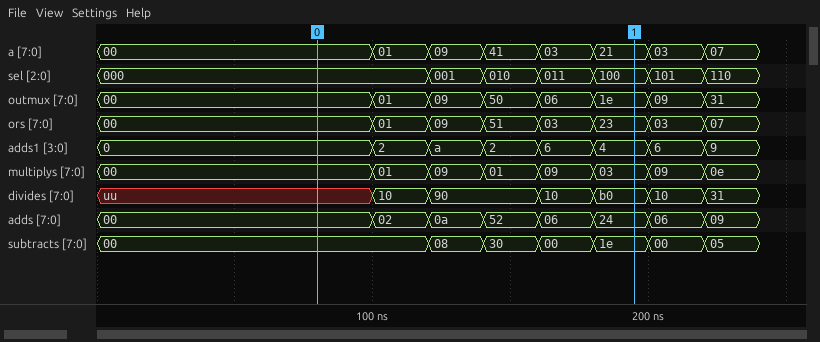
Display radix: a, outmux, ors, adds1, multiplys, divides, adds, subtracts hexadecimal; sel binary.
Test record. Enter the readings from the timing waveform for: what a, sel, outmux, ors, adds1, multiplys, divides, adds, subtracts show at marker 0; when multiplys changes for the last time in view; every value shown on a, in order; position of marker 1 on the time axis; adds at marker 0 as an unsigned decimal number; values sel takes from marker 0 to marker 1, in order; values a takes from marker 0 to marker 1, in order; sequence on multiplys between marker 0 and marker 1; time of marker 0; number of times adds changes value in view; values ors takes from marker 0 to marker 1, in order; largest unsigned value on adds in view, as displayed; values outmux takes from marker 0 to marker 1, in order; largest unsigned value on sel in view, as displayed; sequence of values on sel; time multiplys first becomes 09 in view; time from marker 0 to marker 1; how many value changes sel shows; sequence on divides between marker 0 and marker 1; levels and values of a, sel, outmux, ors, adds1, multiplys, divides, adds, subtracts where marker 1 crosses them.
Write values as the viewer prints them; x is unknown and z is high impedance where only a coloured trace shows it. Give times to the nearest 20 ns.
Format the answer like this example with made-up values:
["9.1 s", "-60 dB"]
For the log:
["a=00, sel=000, outmux=00, ors=00, adds1=0, multiplys=00, divides=uu, adds=00, subtracts=00", "220 ns", "00, 01, 09, 41, 03, 21, 03, 07", "200 ns", "0", "000, 001, 010, 011, 100", "00, 01, 09, 41, 03, 21", "00, 01, 09, 01, 09, 03", "80 ns", "7", "00, 01, 09, 51, 03, 23", "52", "00, 01, 09, 50, 06, 1e", "110", "000, 001, 010, 011, 100, 101, 110", "120 ns", "120 ns", "6", "uu, 10, 90, 10, b0", "a=21, sel=100, outmux=1e, ors=23, adds1=4, multiplys=03, divides=b0, adds=24, subtracts=1e"]
